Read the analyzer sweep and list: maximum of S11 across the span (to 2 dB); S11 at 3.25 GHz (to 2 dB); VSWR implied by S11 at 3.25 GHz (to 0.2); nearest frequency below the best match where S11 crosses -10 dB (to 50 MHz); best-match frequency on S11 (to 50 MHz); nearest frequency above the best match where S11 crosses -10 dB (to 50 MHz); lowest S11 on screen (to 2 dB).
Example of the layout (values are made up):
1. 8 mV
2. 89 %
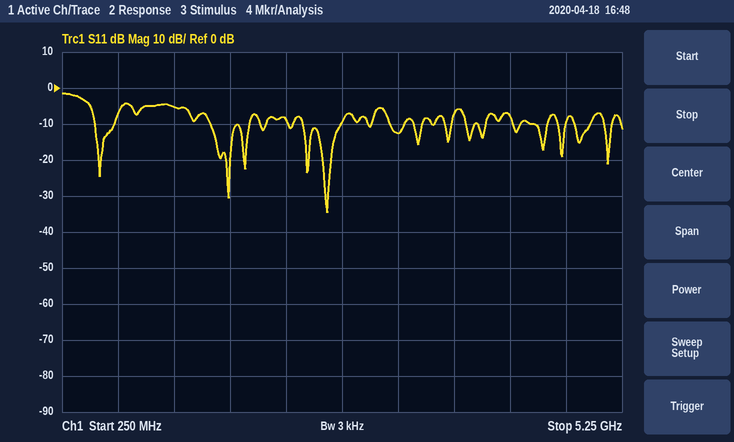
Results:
1. -2 dB
2. -12 dB
3. 1.6
4. 2.40 GHz
5. 2.60 GHz
6. 2.75 GHz
7. -34 dB
